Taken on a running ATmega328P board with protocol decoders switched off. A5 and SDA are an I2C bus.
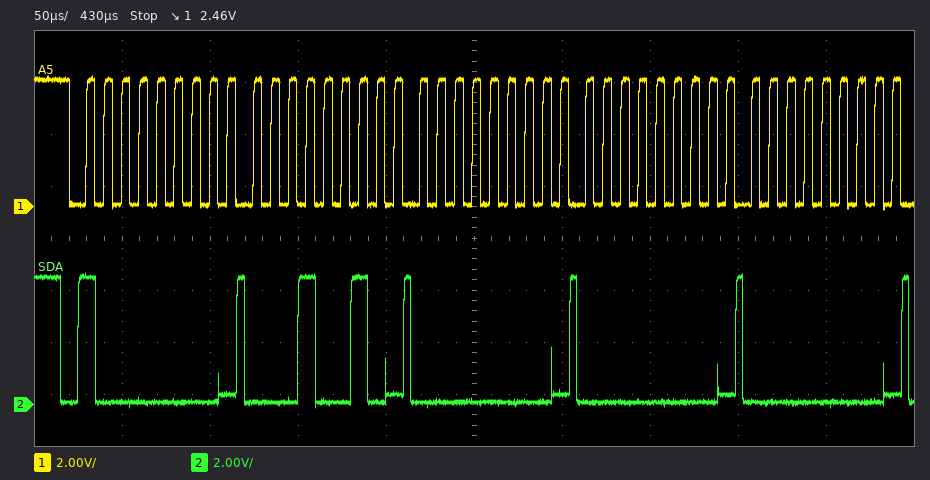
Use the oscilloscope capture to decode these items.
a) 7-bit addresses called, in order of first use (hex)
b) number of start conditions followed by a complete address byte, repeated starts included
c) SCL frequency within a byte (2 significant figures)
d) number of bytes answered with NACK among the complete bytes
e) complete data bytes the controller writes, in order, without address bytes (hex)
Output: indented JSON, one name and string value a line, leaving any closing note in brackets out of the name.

{
  "7-bit addresses called, in order of first use": "0x40",
  "number of start conditions followed by a complete address byte, repeated starts included": "1",
  "SCL frequency within a byte": "100 kHz",
  "number of bytes answered with NACK among the complete bytes": "0",
  "complete data bytes the controller writes, in order, without address bytes": "12 00 00 00"
}
